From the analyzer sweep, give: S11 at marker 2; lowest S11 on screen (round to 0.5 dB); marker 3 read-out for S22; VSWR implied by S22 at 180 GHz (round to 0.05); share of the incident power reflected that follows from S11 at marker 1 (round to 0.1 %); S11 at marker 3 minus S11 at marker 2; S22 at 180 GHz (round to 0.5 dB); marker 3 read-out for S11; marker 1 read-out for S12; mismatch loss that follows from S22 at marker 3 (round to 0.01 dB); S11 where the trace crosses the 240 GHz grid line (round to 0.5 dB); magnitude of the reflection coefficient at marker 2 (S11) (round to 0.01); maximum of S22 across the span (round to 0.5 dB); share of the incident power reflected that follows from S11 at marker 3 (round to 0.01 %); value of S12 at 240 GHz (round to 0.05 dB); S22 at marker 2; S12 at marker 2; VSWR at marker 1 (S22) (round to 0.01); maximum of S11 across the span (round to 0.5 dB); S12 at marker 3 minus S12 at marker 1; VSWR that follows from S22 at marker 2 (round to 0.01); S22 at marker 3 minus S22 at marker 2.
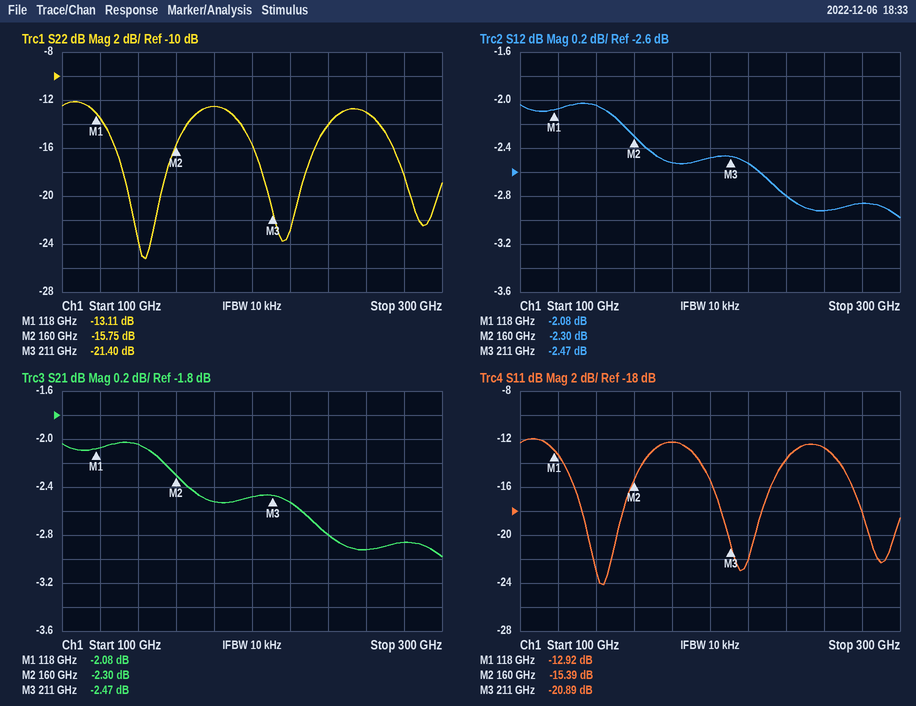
-15.39 dB
-24.0 dB
-21.40 dB
1.60
5.1 %
-5.50 dB
-12.5 dB
-20.89 dB
-2.08 dB
0.03 dB
-13.5 dB
0.17
-12.0 dB
0.81 %
-2.80 dB
-15.75 dB
-2.30 dB
1.57
-12.0 dB
-0.39 dB
1.39
-5.65 dB
